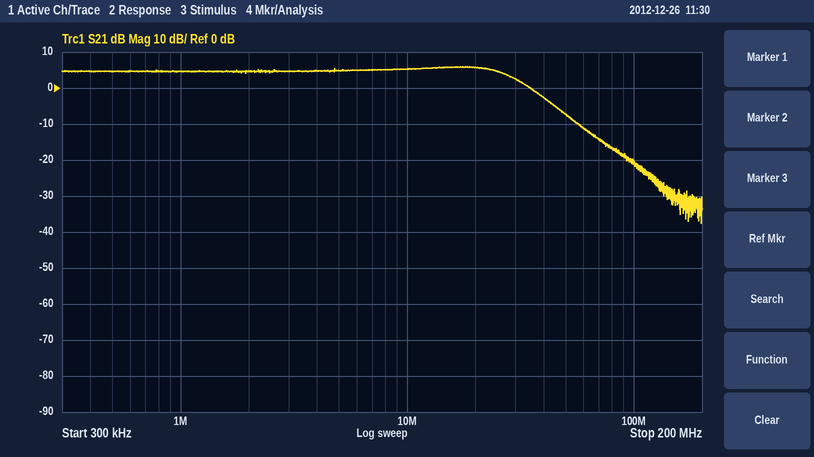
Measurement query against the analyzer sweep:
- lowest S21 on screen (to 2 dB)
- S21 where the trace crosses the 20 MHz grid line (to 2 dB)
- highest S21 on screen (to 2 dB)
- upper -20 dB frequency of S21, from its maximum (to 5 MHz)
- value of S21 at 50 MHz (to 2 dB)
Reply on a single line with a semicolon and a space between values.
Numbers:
-38 dB; 6 dB; 6 dB; 70 MHz; -8 dB
